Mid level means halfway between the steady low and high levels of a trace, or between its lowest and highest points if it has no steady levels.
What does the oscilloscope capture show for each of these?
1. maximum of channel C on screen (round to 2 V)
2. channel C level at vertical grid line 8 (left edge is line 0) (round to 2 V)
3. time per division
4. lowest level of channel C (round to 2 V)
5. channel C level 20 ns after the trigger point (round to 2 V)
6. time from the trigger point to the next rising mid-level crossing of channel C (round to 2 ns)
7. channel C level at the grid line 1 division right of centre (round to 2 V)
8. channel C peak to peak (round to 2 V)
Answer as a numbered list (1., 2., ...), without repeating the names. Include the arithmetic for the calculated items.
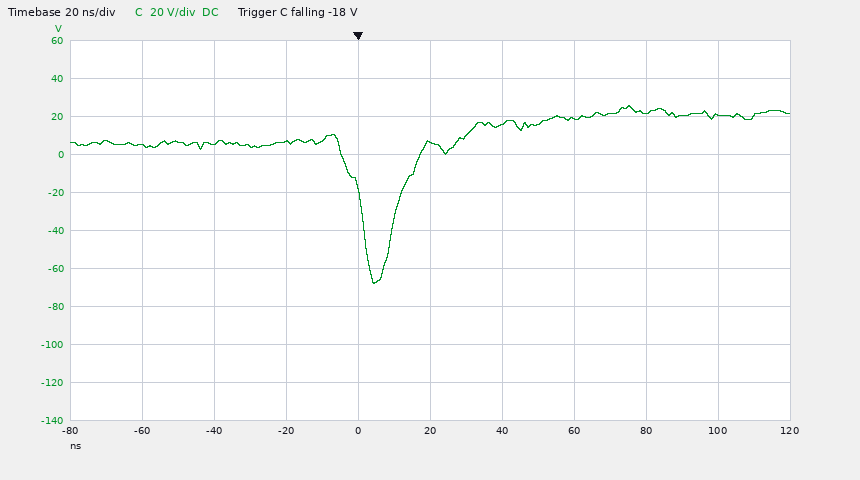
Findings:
1. 26 V
2. 22 V
3. 20 ns
4. -68 V
5. 6 V
6. 12 ns
7. 16 V
8. 26 V − (-68 V) = 94 V
